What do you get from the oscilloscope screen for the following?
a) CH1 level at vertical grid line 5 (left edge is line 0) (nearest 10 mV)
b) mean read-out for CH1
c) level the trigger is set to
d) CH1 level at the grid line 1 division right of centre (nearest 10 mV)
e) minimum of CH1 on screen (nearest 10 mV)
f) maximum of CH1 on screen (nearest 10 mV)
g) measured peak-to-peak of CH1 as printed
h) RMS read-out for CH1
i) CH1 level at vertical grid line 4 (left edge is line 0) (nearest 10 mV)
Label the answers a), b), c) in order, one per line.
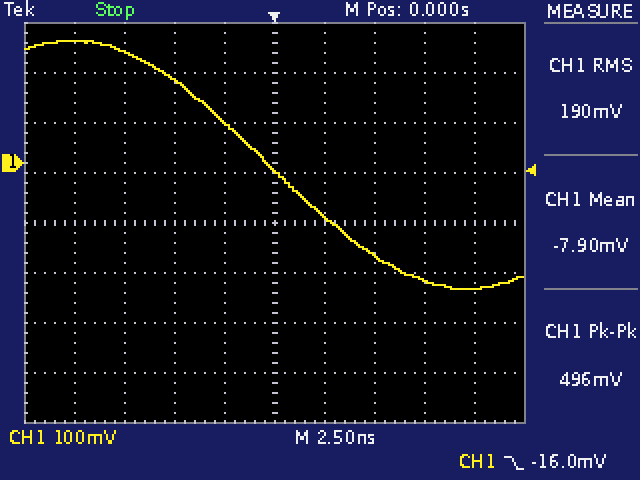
a) -10 mV
b) -7.90 mV
c) -16.0 mV
d) -110 mV
e) -250 mV
f) 240 mV
g) 496 mV
h) 190 mV
i) 80 mV
